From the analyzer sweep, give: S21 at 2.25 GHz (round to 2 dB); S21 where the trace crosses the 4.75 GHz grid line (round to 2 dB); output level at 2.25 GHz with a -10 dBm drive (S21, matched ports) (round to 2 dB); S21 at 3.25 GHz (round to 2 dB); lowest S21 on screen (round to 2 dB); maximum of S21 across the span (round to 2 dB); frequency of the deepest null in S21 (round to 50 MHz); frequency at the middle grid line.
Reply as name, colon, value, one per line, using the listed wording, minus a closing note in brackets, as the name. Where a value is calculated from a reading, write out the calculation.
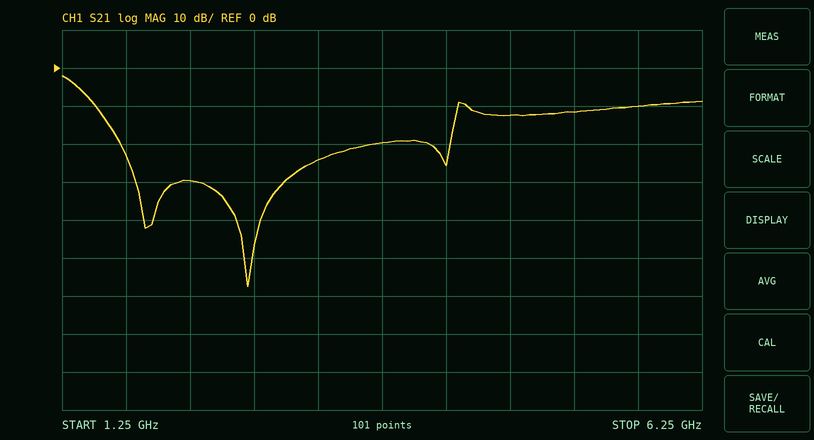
S21 at 2.25 GHz: -30 dB
S21 where the trace crosses the 4.75 GHz grid line: -12 dB
output level at 2.25 GHz with a -10 dBm drive (S21, matched ports): -10 dBm + (-30 dB) = -40 dBm
S21 at 3.25 GHz: -24 dB
lowest S21 on screen: -58 dB
maximum of S21 across the span: -2 dB
frequency of the deepest null in S21: 2.70 GHz
frequency at the middle grid line: 3.75 GHz
